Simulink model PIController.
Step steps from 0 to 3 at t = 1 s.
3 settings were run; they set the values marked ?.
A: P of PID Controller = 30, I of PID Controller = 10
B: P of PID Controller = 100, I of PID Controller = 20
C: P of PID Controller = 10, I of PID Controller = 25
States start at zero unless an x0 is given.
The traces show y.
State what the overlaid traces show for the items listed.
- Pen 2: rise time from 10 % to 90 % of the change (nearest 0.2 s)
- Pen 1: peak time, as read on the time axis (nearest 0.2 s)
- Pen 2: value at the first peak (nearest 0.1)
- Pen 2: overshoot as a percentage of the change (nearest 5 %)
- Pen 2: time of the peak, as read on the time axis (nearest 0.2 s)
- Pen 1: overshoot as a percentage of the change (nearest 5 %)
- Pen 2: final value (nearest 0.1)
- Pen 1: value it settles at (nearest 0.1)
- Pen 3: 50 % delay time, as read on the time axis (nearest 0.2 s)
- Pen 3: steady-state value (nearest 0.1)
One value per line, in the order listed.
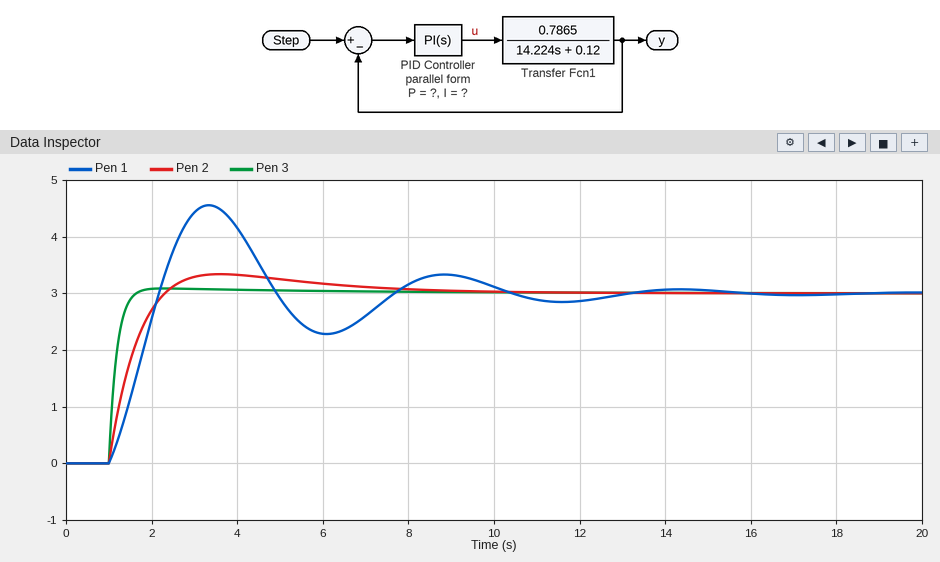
1.0 s
3.4 s
3.3
10 %
3.6 s
50 %
3.0
3.0
1.2 s
3.0
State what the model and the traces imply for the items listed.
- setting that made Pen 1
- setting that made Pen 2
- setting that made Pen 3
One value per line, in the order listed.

C
A
B
